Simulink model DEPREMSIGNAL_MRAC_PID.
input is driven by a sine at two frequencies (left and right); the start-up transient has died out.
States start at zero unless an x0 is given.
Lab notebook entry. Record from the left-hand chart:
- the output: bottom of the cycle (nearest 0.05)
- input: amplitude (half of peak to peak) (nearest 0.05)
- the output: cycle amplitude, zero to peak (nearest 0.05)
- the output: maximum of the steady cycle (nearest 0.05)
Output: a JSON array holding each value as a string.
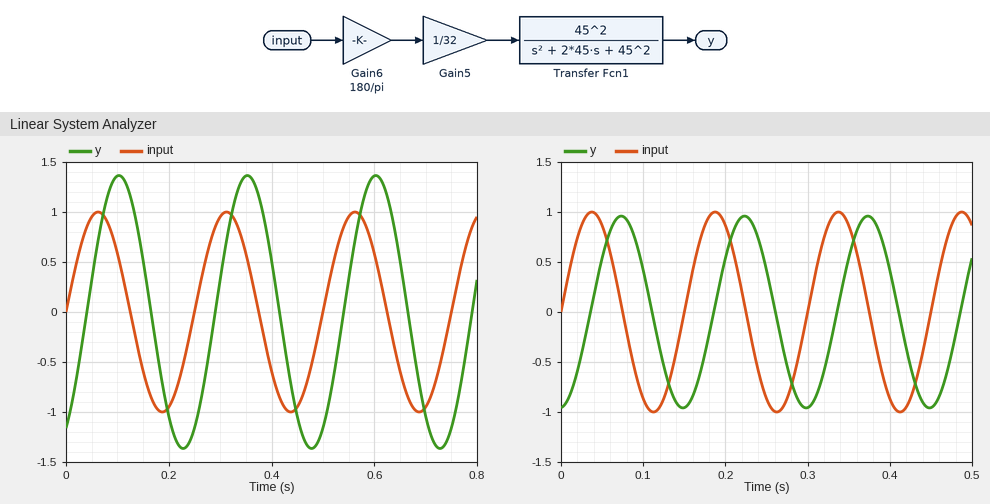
["-1.35", "1.00", "1.35", "1.35"]
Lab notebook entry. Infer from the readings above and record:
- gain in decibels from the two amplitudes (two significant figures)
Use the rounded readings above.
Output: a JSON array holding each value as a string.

["2.6 dB"]
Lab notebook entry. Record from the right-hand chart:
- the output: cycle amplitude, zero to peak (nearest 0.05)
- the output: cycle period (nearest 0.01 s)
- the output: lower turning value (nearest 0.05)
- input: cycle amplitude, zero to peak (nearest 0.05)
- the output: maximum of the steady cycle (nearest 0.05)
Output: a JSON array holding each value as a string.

["0.95", "0.15 s", "-0.95", "1.00", "0.95"]
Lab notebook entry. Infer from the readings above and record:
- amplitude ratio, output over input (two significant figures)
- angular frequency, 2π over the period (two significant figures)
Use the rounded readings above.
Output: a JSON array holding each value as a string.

["0.95", "42 rad/s"]
